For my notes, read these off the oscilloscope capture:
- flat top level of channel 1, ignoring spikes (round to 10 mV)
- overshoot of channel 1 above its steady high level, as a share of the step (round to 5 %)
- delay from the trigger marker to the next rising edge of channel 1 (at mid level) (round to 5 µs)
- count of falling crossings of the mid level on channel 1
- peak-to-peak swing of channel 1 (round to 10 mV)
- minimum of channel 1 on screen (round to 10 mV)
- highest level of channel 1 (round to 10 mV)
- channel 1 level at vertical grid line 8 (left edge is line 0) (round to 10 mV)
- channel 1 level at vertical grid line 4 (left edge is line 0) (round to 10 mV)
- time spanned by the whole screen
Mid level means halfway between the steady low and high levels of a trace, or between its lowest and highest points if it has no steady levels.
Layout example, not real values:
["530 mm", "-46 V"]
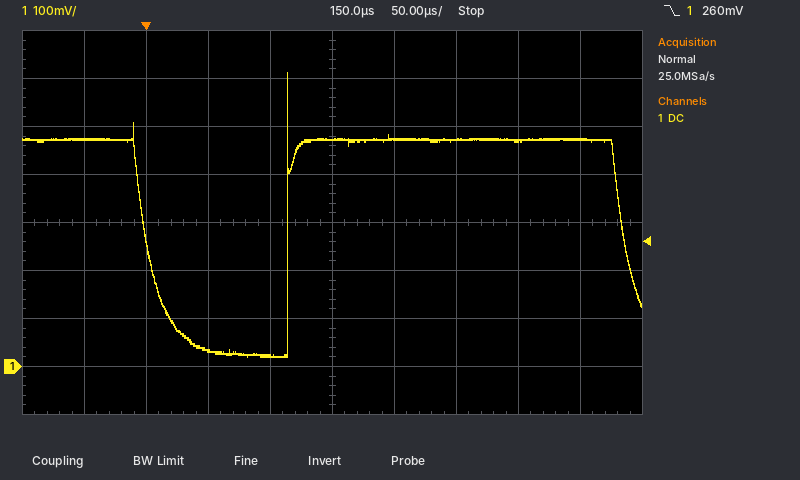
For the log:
["470 mV", "30 %", "115 µs", "2", "590 mV", "20 mV", "610 mV", "470 mV", "20 mV", "500 µs"]
